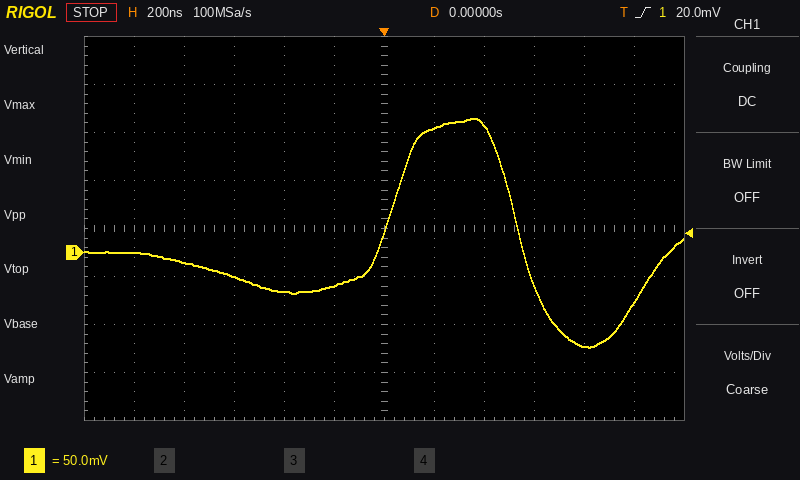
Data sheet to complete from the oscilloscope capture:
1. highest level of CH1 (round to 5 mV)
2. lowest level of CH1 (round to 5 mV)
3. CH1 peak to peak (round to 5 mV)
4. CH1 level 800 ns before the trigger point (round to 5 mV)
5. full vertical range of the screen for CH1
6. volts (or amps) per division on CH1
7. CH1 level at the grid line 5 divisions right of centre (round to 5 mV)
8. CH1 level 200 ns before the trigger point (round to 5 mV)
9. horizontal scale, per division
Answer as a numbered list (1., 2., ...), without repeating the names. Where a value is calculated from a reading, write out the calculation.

1. 140 mV
2. -100 mV
3. 140 mV − (-100 mV) = 240 mV
4. -10 mV
5. 400 mV
6. 50 mV
7. -50 mV
8. -35 mV
9. 200 ns
